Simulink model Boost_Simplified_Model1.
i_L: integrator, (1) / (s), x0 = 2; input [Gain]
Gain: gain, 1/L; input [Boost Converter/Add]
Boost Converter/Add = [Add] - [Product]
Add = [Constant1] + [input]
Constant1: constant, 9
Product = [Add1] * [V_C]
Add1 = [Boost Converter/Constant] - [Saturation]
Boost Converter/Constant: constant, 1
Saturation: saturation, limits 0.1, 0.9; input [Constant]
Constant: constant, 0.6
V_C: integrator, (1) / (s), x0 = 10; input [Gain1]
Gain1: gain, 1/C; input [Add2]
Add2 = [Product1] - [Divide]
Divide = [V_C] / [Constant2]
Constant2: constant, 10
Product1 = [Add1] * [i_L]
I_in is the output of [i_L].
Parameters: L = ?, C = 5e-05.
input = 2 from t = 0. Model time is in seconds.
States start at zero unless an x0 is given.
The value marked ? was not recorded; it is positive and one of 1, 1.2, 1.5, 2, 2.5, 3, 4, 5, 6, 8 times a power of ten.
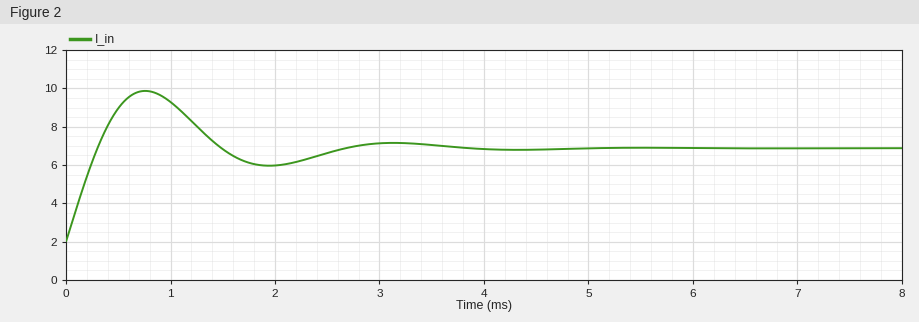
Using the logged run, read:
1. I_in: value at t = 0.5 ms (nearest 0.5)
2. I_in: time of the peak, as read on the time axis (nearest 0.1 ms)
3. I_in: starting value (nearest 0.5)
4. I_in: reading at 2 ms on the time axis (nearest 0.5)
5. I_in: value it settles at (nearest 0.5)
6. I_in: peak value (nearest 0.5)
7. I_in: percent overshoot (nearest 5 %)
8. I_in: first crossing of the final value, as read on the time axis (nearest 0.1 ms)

9.0
0.8 ms
2.0
6.0
7.0
10.0
60 %
0.3 ms
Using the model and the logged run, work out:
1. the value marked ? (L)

0.0004
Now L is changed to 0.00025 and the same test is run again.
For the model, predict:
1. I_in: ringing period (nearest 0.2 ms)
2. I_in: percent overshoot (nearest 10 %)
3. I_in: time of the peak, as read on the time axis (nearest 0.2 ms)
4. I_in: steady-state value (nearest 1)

1.8 ms
90 %
0.6 ms
7
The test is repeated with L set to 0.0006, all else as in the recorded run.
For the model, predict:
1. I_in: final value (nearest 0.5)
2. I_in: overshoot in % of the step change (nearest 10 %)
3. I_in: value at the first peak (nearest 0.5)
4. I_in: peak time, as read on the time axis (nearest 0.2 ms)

7.0
40 %
9.0
1.0 ms
